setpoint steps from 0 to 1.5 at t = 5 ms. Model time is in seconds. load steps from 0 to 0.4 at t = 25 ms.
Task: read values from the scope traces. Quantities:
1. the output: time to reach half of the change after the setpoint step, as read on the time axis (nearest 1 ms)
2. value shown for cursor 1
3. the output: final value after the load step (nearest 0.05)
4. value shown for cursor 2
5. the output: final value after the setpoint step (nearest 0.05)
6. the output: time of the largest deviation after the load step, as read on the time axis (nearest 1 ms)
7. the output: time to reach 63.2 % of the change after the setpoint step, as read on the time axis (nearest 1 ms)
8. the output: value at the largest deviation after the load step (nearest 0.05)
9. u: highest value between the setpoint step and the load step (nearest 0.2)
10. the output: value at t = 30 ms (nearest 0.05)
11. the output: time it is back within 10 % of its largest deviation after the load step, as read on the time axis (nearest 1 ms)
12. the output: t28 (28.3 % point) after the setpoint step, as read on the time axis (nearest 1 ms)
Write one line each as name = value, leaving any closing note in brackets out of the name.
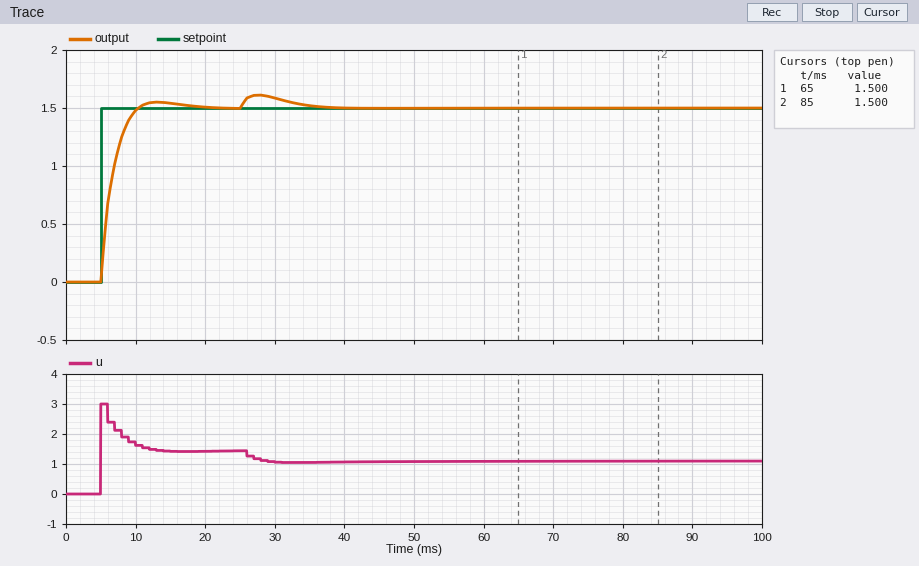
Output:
the output: time to reach half of the change after the setpoint step, as read on the time axis = 6 ms
value shown for cursor 1 = 1.500
the output: final value after the load step = 1.50
value shown for cursor 2 = 1.500
the output: final value after the setpoint step = 1.50
the output: time of the largest deviation after the load step, as read on the time axis = 28 ms
the output: time to reach 63.2 % of the change after the setpoint step, as read on the time axis = 7 ms
the output: value at the largest deviation after the load step = 1.60
u: highest value between the setpoint step and the load step = 3.0
the output: value at t = 30 ms = 1.60
the output: time it is back within 10 % of its largest deviation after the load step, as read on the time axis = 36 ms
the output: t28 (28.3 % point) after the setpoint step, as read on the time axis = 6 ms
